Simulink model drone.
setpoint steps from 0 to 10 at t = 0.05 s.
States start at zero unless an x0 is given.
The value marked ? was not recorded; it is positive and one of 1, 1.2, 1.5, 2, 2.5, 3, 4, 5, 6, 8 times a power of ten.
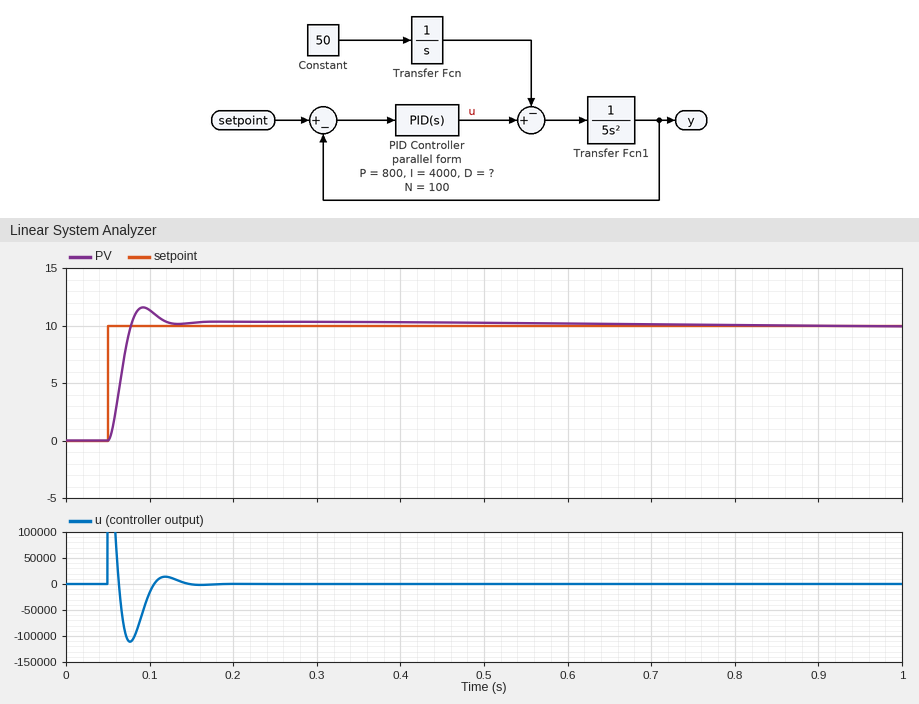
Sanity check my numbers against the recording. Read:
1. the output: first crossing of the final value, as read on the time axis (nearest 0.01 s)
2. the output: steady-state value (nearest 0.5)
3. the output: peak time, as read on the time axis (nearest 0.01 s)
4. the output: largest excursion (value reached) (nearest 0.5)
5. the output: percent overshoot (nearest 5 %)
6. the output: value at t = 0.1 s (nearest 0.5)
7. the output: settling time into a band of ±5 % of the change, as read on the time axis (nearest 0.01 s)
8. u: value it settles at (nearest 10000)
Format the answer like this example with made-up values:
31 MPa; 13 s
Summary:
0.08 s; 10.0; 0.09 s; 11.5; 15 %; 11.5; 0.12 s; 0
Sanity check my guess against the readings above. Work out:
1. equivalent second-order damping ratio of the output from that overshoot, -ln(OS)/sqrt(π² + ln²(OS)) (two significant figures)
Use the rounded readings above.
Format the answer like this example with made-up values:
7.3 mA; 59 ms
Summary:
0.52
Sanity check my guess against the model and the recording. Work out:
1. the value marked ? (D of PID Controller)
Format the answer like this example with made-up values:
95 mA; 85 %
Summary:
400
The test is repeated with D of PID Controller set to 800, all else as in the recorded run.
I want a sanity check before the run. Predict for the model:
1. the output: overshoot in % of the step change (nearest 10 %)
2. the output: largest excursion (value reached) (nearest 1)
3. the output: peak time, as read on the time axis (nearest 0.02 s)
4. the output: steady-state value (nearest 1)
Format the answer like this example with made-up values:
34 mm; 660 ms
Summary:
30 %; 13; 0.08 s; 10
